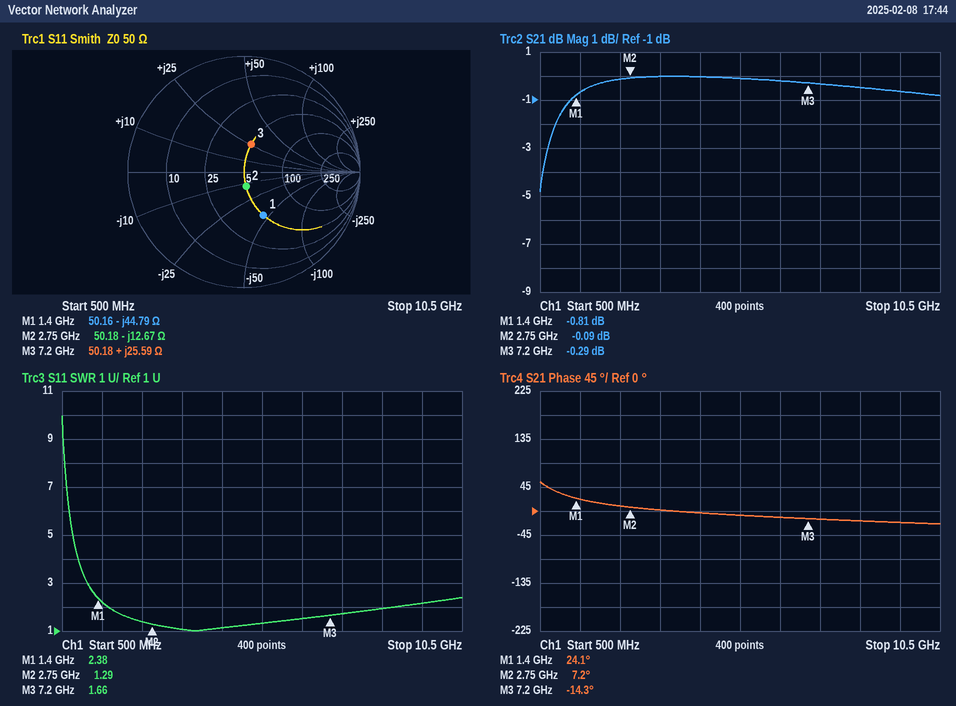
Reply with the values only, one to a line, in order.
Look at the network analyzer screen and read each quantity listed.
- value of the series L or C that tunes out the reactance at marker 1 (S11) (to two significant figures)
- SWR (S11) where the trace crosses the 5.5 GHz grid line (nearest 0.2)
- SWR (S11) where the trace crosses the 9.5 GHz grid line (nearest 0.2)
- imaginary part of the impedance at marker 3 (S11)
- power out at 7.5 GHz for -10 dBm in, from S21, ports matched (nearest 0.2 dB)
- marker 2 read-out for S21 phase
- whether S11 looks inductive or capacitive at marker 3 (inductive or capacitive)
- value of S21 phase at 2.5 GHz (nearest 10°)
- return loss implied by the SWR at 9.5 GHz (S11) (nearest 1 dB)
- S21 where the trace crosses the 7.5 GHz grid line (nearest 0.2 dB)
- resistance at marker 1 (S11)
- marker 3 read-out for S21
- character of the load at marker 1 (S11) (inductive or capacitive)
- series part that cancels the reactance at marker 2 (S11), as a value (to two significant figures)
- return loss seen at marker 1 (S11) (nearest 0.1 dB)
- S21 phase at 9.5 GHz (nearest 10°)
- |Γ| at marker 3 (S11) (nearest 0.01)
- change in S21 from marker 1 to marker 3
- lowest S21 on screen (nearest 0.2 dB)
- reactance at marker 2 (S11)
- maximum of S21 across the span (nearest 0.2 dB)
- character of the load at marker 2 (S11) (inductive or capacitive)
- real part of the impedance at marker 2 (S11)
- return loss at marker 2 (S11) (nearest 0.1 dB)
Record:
5.1 nH
1.4
2.2
+25.59 Ω
-10.4 dBm
7.2°
inductive
10°
9 dB
-0.4 dB
50.16 Ω
-0.29 dB
capacitive
730 pH
7.8 dB
-20°
0.25
0.52 dB
-4.8 dB
-12.67 Ω
0.0 dB
capacitive
50.18 Ω
18.0 dB
